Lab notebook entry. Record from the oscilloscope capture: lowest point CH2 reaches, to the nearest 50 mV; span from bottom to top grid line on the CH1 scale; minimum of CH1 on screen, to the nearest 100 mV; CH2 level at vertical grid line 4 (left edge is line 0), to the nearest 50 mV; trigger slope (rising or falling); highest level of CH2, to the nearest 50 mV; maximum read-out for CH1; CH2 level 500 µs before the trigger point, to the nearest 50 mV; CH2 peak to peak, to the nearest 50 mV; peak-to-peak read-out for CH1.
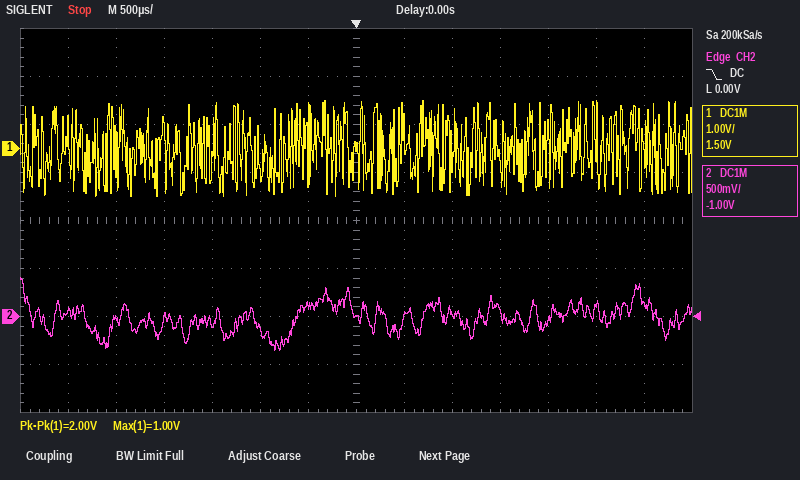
-350 mV
8 V
-1.0 V
-50 mV
falling
400 mV
1.00 V
100 mV
750 mV
2.00 V
